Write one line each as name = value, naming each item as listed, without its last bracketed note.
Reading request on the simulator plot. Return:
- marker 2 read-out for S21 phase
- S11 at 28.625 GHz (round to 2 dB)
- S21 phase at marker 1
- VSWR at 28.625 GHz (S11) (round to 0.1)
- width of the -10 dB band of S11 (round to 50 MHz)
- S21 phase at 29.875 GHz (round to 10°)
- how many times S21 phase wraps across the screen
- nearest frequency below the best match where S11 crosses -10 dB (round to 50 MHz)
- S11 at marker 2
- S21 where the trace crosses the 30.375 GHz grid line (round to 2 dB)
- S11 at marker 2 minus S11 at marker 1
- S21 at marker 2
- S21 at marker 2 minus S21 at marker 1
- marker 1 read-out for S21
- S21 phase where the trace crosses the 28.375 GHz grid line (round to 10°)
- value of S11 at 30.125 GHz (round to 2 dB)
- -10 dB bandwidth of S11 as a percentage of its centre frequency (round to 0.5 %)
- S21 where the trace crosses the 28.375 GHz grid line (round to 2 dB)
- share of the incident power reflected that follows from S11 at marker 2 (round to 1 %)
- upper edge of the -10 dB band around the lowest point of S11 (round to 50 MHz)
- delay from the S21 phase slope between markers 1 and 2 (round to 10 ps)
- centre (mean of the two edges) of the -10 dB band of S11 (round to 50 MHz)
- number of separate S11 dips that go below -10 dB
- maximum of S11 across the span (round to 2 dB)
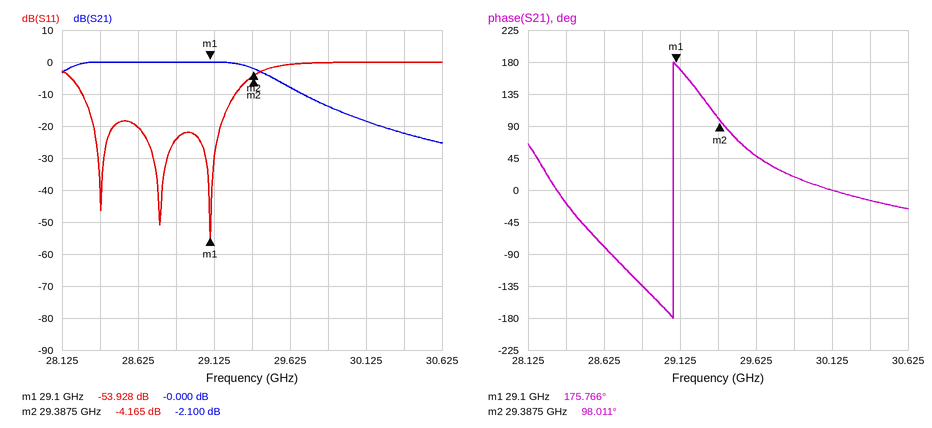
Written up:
marker 2 read-out for S21 phase = 98.011°
S11 at 28.625 GHz = -20 dB
S21 phase at marker 1 = 175.766°
VSWR at 28.625 GHz (S11) = 1.2
width of the -10 dB band of S11 = 1.00 GHz
S21 phase at 29.875 GHz = 20°
how many times S21 phase wraps across the screen = 1
nearest frequency below the best match where S11 crosses -10 dB = 28.25 GHz
S11 at marker 2 = -4.165 dB
S21 where the trace crosses the 30.375 GHz grid line = -22 dB
S11 at marker 2 minus S11 at marker 1 = 49.763 dB
S21 at marker 2 = -2.100 dB
S21 at marker 2 minus S21 at marker 1 = -2.100 dB
marker 1 read-out for S21 = -0.000 dB
S21 phase where the trace crosses the 28.375 GHz grid line = -20°
value of S11 at 30.125 GHz = 0 dB
-10 dB bandwidth of S11 as a percentage of its centre frequency = 3.5 %
S21 where the trace crosses the 28.375 GHz grid line = 0 dB
share of the incident power reflected that follows from S11 at marker 2 = 38 %
upper edge of the -10 dB band around the lowest point of S11 = 29.25 GHz
delay from the S21 phase slope between markers 1 and 2 = 750 ps
centre (mean of the two edges) of the -10 dB band of S11 = 28.75 GHz
number of separate S11 dips that go below -10 dB = 3
maximum of S11 across the span = 0 dB
